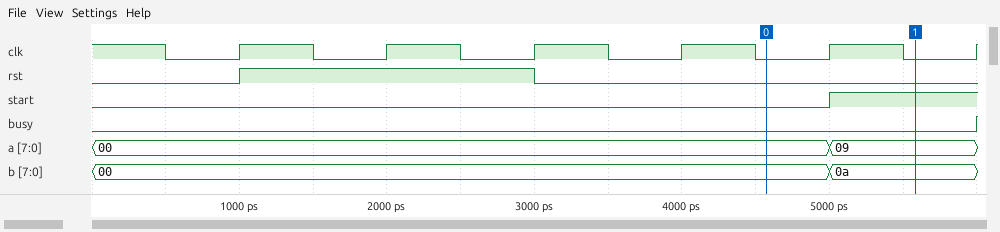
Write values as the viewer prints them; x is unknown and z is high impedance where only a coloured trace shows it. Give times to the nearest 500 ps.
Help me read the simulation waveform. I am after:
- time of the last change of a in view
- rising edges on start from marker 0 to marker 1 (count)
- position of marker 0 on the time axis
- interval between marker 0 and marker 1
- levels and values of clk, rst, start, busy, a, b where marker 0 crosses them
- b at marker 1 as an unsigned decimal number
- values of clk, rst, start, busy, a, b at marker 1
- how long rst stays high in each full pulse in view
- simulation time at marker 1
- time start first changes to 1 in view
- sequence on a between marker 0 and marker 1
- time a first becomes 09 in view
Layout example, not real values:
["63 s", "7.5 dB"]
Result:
["5000 ps", "1", "4500 ps", "1000 ps", "clk=0, rst=0, start=0, busy=0, a=00, b=00", "10", "clk=0, rst=0, start=1, busy=0, a=09, b=0a", "2000 ps", "5500 ps", "5000 ps", "00, 09", "5000 ps"]
